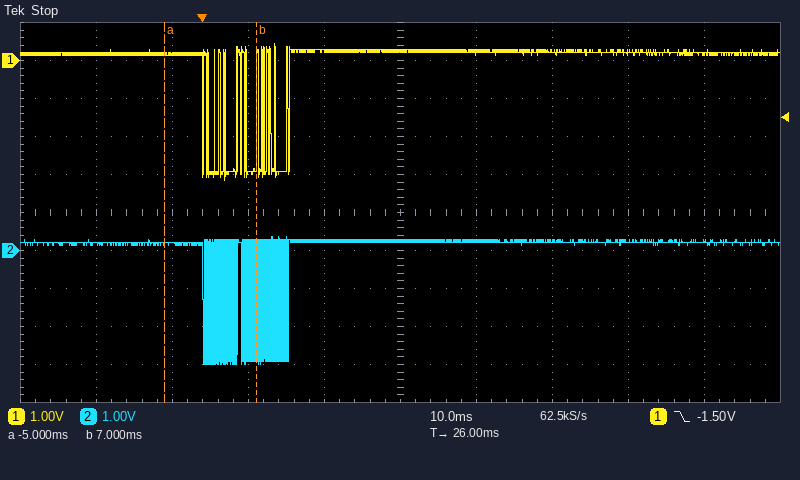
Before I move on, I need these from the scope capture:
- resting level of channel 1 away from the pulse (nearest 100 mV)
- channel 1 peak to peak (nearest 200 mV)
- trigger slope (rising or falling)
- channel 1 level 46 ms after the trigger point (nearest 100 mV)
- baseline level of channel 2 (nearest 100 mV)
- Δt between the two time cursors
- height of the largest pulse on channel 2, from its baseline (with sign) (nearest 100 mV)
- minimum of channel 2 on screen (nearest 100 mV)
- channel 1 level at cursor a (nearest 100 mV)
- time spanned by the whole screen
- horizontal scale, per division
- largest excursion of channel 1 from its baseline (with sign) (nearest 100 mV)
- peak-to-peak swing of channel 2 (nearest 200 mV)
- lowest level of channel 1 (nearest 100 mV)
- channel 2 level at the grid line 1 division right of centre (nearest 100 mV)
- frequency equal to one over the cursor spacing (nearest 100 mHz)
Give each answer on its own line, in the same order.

200 mV
3.6 V
falling
200 mV
200 mV
12 ms
-3.2 V
-3.0 V
200 mV
100 ms
10 ms
-3.4 V
3.4 V
-3.2 V
200 mV
83.3 Hz
